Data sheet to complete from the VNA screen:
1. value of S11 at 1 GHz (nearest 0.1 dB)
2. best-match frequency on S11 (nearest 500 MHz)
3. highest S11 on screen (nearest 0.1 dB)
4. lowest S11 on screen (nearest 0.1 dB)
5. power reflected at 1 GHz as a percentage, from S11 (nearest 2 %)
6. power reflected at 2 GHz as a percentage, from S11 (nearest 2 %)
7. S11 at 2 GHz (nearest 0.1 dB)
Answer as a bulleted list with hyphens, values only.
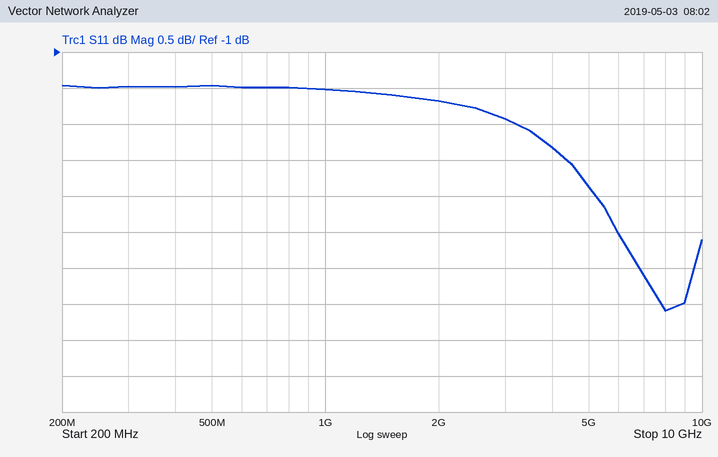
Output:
- -1.5 dB
- 8.0 GHz
- -1.5 dB
- -4.6 dB
- 70 %
- 68 %
- -1.7 dB
